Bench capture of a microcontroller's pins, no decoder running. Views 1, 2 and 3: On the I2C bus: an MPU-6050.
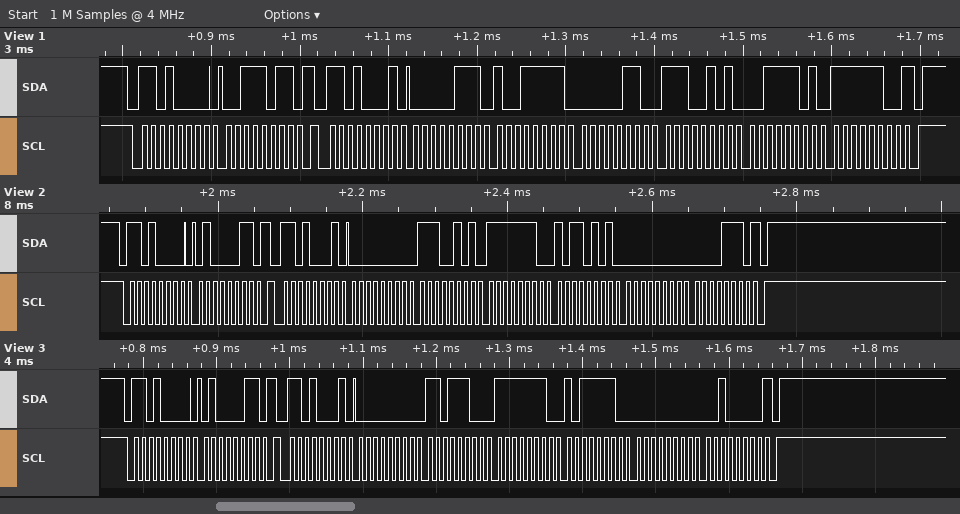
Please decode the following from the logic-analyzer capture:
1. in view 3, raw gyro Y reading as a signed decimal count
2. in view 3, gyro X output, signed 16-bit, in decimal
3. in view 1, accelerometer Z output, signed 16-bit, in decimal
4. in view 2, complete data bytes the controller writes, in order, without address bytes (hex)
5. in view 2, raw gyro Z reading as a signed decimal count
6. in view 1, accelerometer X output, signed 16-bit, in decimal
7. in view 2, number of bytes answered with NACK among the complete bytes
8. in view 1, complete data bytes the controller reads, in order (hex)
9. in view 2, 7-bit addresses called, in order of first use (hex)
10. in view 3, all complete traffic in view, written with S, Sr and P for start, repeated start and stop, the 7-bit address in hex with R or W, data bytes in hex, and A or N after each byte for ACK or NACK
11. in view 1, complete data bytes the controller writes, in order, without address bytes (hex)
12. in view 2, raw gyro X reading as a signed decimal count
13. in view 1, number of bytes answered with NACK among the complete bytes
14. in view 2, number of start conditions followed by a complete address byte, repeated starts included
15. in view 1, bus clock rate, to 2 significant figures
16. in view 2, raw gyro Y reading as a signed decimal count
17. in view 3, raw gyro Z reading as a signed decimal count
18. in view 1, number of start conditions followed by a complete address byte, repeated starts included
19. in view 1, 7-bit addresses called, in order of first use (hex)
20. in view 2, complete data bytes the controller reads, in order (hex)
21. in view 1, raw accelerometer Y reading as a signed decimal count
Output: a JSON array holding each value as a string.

["-322", "220", "15868", "43", "14", "1951", "1", "07 9F 06 E5 3D FC", "0x68", "S 68W A 43 A Sr 68R A 00 A DC A FE A BE A 00 A 20 N P", "3B", "229", "1", "2", "100 kHz", "-331", "32", "2", "0x68", "00 E5 FE B5 00 0E", "1765"]
